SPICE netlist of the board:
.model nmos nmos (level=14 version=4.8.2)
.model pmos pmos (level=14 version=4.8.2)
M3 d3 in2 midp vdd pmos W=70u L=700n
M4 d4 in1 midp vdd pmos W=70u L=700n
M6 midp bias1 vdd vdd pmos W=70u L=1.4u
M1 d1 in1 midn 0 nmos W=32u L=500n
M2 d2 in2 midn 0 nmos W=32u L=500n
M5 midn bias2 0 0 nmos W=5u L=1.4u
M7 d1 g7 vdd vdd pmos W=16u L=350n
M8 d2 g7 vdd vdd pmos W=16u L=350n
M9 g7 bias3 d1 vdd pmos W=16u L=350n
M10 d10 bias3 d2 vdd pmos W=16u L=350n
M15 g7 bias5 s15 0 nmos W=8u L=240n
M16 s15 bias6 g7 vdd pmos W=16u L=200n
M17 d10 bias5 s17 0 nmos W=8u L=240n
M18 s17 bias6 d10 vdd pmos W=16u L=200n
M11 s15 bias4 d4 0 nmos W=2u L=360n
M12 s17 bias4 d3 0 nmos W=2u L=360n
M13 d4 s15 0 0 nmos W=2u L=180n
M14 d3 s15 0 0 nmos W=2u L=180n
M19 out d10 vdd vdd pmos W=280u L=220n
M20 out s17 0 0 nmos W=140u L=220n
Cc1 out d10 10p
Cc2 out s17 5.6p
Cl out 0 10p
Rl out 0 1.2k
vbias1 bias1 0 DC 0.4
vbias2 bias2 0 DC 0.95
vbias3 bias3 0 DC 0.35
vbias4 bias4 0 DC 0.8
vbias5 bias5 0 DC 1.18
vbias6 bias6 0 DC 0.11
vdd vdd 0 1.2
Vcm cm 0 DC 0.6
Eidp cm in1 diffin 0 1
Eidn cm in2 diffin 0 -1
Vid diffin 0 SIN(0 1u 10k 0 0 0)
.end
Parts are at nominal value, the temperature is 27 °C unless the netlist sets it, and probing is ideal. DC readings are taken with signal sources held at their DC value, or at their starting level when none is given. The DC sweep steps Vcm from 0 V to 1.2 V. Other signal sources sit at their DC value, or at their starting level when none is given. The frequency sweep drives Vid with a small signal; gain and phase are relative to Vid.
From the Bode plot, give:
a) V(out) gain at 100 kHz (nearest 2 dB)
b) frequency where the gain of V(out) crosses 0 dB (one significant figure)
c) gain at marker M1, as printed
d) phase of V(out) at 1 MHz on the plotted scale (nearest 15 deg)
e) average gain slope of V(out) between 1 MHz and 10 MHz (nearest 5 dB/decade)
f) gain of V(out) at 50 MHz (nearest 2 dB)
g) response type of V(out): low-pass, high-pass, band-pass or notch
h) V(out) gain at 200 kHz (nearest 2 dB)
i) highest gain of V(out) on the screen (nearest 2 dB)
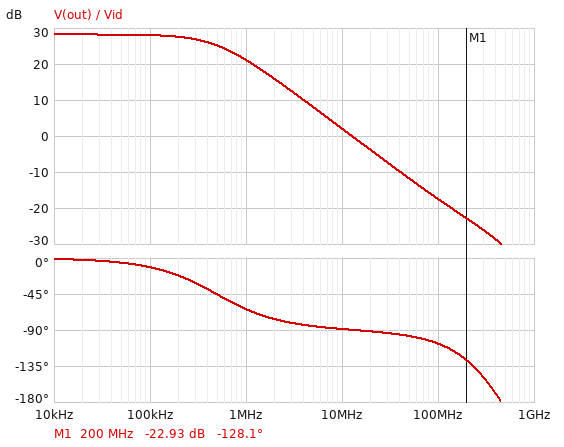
28 dB
10 MHz
-22.93 dB
-60 deg
-20 dB/decade
-12 dB
low-pass
28 dB
28 dB
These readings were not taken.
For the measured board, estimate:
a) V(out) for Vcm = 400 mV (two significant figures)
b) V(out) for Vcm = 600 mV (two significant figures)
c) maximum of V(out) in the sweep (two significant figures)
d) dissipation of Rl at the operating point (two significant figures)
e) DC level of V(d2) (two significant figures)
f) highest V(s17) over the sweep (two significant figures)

12 mV
26 mV
130 mV
570 nW
790 mV
1.1 V
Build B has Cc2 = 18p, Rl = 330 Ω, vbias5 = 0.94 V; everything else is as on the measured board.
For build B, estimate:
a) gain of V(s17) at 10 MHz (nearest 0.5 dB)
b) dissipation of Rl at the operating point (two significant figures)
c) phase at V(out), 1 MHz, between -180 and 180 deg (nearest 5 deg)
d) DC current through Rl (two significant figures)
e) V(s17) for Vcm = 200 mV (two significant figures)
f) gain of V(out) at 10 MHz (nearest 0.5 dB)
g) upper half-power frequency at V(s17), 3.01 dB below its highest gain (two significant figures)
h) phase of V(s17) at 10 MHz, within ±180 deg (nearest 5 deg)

5.5 dB
2.0 µW
-75 deg
78 µA
930 mV
-2.5 dB
290 kHz
80 deg
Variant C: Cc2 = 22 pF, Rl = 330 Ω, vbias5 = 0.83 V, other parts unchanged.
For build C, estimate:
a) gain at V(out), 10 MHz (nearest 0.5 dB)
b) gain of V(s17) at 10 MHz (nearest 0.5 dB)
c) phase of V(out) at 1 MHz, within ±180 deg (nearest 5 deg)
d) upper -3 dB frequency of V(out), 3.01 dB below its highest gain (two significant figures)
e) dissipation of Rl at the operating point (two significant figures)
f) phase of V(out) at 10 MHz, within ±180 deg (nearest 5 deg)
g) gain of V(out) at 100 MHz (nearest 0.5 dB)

-3.5 dB
4.5 dB
-75 deg
250 kHz
2.0 µW
-85 deg
-18.5 dB
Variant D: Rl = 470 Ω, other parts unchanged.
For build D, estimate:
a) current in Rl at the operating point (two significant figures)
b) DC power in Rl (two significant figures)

55 µA
1.4 µW
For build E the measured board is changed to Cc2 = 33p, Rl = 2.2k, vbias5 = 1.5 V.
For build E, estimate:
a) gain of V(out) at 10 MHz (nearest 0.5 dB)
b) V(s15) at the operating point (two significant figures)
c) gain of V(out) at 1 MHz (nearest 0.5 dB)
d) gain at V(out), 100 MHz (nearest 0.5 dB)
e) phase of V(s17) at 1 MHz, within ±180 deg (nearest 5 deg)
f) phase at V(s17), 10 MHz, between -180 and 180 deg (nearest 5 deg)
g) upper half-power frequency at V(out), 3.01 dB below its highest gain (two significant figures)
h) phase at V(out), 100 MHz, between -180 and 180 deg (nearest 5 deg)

-6.0 dB
790 mV
13.5 dB
-22.0 dB
100 deg
85 deg
190 kHz
-85 deg
